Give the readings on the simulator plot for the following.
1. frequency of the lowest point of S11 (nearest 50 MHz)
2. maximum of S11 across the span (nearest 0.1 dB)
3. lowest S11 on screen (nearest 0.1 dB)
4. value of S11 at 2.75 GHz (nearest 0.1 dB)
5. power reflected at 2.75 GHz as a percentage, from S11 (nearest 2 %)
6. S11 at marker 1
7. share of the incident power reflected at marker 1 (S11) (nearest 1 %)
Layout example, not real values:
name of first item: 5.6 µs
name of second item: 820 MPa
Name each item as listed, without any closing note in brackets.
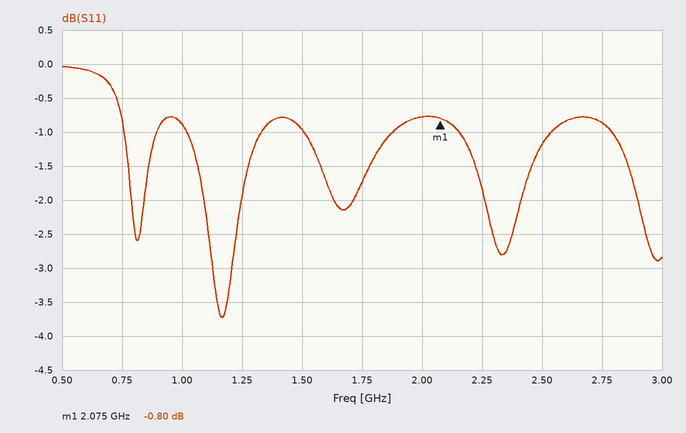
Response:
frequency of the lowest point of S11: 1.15 GHz
maximum of S11 across the span: 0.0 dB
lowest S11 on screen: -3.7 dB
value of S11 at 2.75 GHz: -0.9 dB
power reflected at 2.75 GHz as a percentage, from S11: 82 %
S11 at marker 1: -0.80 dB
share of the incident power reflected at marker 1 (S11): 83 %
